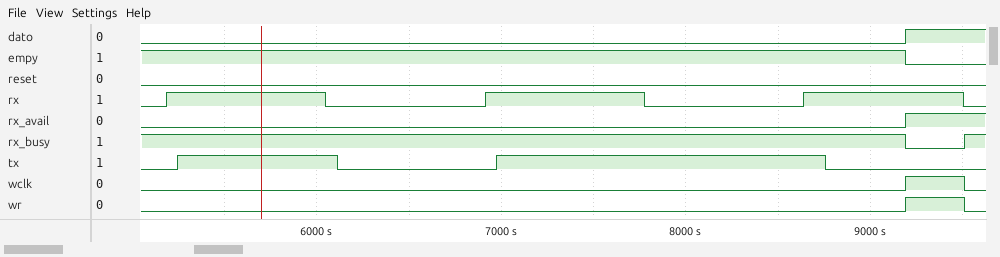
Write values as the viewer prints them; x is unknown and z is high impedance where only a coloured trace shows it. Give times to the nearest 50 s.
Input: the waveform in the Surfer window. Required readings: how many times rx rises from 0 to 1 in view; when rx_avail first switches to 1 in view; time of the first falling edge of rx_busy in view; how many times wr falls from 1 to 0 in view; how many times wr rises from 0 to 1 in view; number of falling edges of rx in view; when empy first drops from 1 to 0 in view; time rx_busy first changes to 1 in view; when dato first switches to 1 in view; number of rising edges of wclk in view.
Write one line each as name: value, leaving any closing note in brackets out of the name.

how many times rx rises from 0 to 1 in view: 3
when rx_avail first switches to 1 in view: 9200 s
time of the first falling edge of rx_busy in view: 9200 s
how many times wr falls from 1 to 0 in view: 1
how many times wr rises from 0 to 1 in view: 1
number of falling edges of rx in view: 3
when empy first drops from 1 to 0 in view: 9200 s
time rx_busy first changes to 1 in view: 9500 s
when dato first switches to 1 in view: 9200 s
number of rising edges of wclk in view: 1
